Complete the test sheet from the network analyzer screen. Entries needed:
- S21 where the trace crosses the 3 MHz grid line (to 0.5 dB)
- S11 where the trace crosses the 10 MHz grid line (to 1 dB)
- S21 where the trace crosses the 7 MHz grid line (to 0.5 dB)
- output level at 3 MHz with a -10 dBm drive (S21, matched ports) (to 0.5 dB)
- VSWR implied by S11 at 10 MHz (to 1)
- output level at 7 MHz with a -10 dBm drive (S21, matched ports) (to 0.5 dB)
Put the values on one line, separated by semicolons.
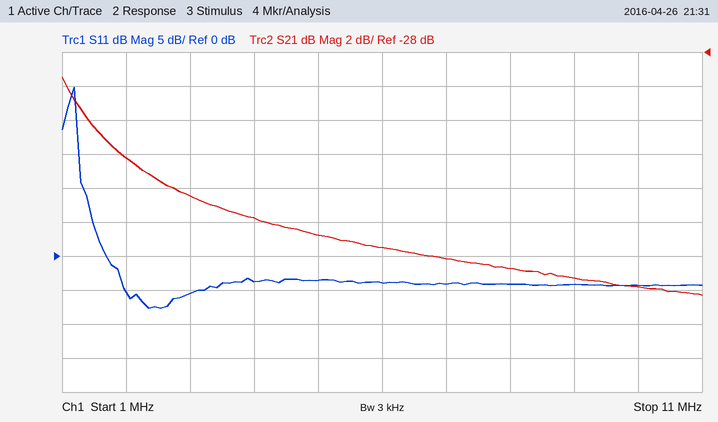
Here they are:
-36.5 dB; -4 dB; -40.0 dB; -46.5 dBm; 4; -50.0 dBm
